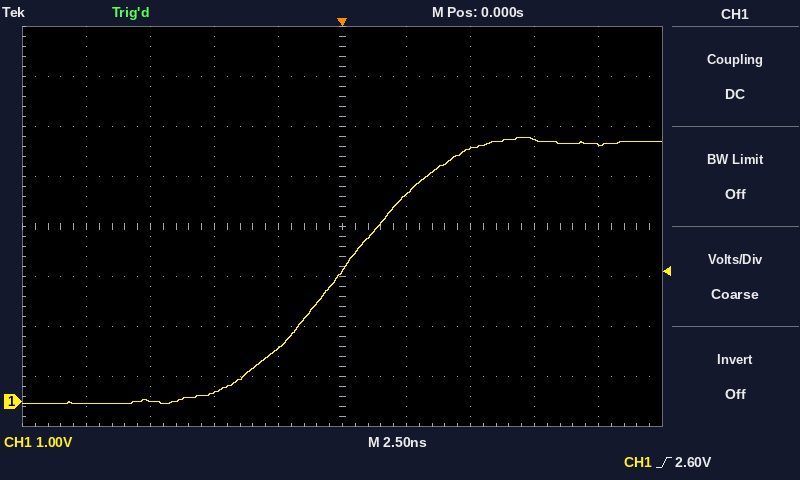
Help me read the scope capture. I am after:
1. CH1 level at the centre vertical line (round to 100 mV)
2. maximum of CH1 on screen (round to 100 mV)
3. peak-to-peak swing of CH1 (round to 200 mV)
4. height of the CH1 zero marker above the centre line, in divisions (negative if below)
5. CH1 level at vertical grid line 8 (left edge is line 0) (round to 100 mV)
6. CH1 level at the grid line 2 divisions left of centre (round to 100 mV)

2.6 V
5.3 V
5.4 V
-3.5 div
5.2 V
200 mV
